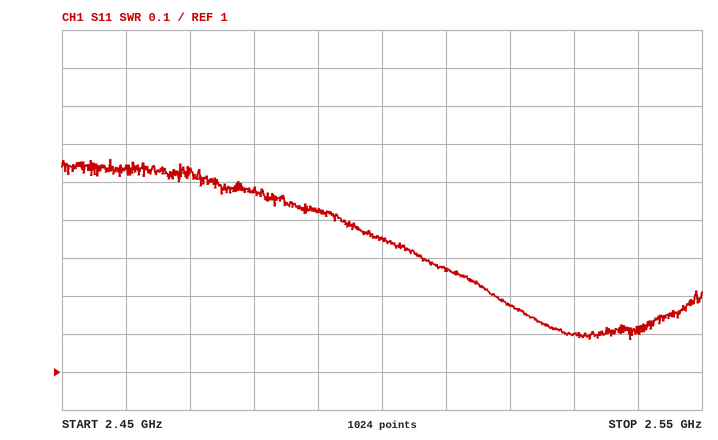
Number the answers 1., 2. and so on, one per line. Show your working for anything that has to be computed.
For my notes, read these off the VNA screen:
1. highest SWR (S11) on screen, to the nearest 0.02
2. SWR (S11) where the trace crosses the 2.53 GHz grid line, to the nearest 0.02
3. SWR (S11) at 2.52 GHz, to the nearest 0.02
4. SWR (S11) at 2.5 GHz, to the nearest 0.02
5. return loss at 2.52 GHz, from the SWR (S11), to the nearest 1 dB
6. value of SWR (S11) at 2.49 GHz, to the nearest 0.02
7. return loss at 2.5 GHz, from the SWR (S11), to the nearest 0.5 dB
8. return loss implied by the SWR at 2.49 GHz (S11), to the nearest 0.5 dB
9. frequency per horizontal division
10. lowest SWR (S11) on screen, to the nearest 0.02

1. 1.56
2. 1.10
3. 1.18
4. 1.36
5. −20 log10((1.18 − 1)/(1.18 + 1)) ≈ 22 dB
6. 1.42
7. −20 log10((1.36 − 1)/(1.36 + 1)) ≈ 16.3 dB, so 16.5 dB to the nearest 0.5 dB
8. −20 log10((1.42 − 1)/(1.42 + 1)) ≈ 15.2 dB, so 15.0 dB to the nearest 0.5 dB
9. 10 MHz
10. 1.08
